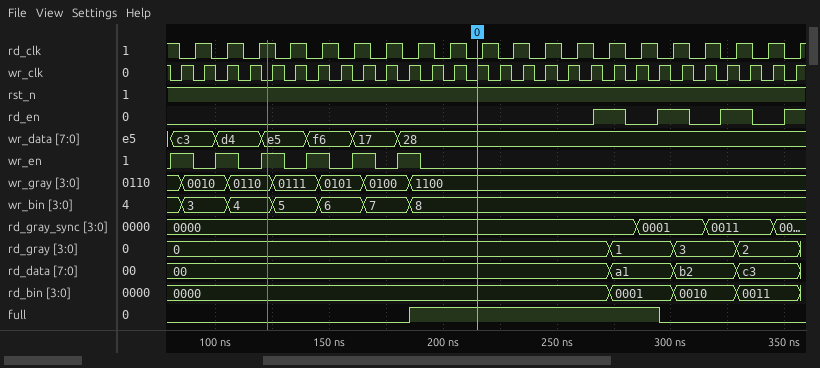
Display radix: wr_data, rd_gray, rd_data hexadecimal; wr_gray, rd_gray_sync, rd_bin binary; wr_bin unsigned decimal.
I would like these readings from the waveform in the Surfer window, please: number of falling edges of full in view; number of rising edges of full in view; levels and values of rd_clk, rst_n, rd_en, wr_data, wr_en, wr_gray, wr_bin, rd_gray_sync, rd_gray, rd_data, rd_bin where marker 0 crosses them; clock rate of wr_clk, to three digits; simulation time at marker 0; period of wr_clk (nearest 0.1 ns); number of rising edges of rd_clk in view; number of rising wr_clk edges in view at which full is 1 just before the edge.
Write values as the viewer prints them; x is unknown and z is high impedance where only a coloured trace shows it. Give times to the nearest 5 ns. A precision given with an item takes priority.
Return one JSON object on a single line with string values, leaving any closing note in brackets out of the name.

{"number of falling edges of full in view": "1", "number of rising edges of full in view": "1", "levels and values of rd_clk, rst_n, rd_en, wr_data, wr_en, wr_gray, wr_bin, rd_gray_sync, rd_gray, rd_data, rd_bin where marker 0 crosses them": "rd_clk=0, rst_n=1, rd_en=0, wr_data=28, wr_en=0, wr_gray=1100, wr_bin=8, rd_gray_sync=0000, rd_gray=0, rd_data=00, rd_bin=0000", "clock rate of wr_clk, to three digits": "100 MHz", "simulation time at marker 0": "215 ns", "period of wr_clk": "10 ns", "number of rising edges of rd_clk in view": "20", "number of rising wr_clk edges in view at which full is 1 just before the edge": "11"}
